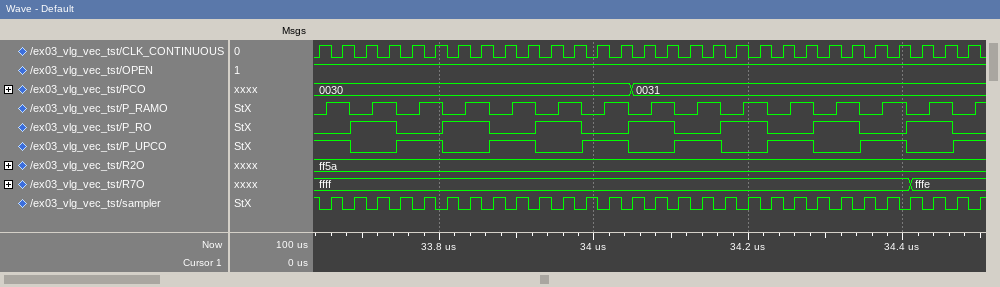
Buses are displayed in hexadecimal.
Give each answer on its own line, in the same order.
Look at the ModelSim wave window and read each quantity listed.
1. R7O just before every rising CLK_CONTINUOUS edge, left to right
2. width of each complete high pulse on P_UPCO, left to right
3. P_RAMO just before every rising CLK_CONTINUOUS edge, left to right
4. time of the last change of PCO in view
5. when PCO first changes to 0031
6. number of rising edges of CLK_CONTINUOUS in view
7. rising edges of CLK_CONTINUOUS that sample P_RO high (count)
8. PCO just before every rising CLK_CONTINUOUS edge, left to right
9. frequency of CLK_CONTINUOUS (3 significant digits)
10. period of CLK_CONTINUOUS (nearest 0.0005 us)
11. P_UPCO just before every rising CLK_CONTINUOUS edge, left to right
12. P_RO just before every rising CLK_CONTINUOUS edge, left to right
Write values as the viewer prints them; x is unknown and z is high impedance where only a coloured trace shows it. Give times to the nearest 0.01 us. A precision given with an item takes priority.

ffff, ffff, ffff, ffff, ffff, ffff, ffff, ffff, ffff, ffff, ffff, ffff, ffff, ffff, ffff, ffff, ffff, ffff, ffff, ffff, ffff, ffff, ffff, ffff, ffff, ffff, fffe, fffe, fffe
0.06 us, 0.06 us, 0.06 us, 0.06 us, 0.06 us, 0.06 us
0 1 0 1 0 1 0 1 0 1 0 1 0 1 0 1 0 1 0 1 0 1 0 1 0 1 0 1 0
34.05 us
34.05 us
29
14
0030, 0030, 0030, 0030, 0030, 0030, 0030, 0030, 0030, 0030, 0030, 0030, 0030, 0030, 0031, 0031, 0031, 0031, 0031, 0031, 0031, 0031, 0031, 0031, 0031, 0031, 0031, 0031, 0031
33.3 MHz
0.03 us
1 1 0 0 1 1 0 0 1 1 0 0 1 1 0 0 1 1 0 0 1 1 0 0 1 1 0 0 1
0 0 1 1 0 0 1 1 0 0 1 1 0 0 1 1 0 0 1 1 0 0 1 1 0 0 1 1 0
